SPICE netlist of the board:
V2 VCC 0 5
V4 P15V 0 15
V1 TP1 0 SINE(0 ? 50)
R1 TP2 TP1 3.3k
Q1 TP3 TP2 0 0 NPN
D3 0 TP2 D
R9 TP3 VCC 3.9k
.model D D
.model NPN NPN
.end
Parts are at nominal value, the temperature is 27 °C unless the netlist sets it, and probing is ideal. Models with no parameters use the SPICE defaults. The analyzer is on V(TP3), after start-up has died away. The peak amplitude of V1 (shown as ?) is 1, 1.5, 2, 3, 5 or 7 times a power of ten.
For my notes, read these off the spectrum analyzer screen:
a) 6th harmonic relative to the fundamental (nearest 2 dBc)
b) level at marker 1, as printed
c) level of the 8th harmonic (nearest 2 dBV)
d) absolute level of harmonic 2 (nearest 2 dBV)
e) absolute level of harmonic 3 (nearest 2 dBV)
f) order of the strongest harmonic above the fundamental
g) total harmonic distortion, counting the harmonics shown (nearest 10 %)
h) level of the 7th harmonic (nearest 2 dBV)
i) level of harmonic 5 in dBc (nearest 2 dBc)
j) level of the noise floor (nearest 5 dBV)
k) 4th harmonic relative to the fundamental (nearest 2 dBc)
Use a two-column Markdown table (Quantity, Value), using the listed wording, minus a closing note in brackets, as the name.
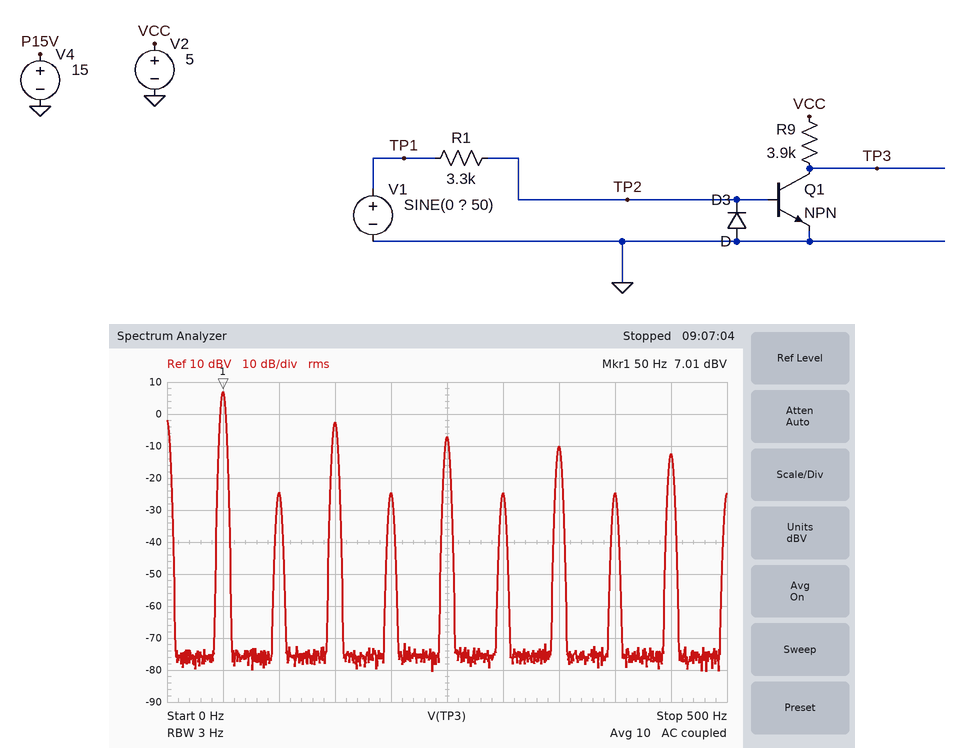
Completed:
| Quantity | Value |
|---|---|
| 6th harmonic relative to the fundamental | -32 dBc |
| level at marker 1, as printed | 7.01 dBV |
| level of the 8th harmonic | -24 dBV |
| absolute level of harmonic 2 | -24 dBV |
| absolute level of harmonic 3 | -2 dBV |
| order of the strongest harmonic above the fundamental | 3 |
| total harmonic distortion, counting the harmonics shown | 40 % |
| level of the 7th harmonic | -10 dBV |
| level of harmonic 5 in dBc | -14 dBc |
| level of the noise floor | -75 dBV |
| 4th harmonic relative to the fundamental | -32 dBc |
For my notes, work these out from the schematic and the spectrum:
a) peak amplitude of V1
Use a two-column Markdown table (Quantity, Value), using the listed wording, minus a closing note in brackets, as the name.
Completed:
| Quantity | Value |
|---|---|
| peak amplitude of V1 | 30 V |
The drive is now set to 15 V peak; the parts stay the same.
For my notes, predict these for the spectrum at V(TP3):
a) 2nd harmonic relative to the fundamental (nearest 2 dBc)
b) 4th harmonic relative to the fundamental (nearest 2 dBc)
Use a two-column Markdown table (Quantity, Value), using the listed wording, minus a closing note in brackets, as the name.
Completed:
| Quantity | Value |
|---|---|
| 2nd harmonic relative to the fundamental | -26 dBc |
| 4th harmonic relative to the fundamental | -26 dBc |
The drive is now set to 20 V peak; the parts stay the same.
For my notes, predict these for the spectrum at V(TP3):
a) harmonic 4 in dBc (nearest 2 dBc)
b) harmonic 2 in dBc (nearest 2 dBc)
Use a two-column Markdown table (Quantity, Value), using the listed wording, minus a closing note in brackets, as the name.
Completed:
| Quantity | Value |
|---|---|
| harmonic 4 in dBc | -28 dBc |
| harmonic 2 in dBc | -28 dBc |
